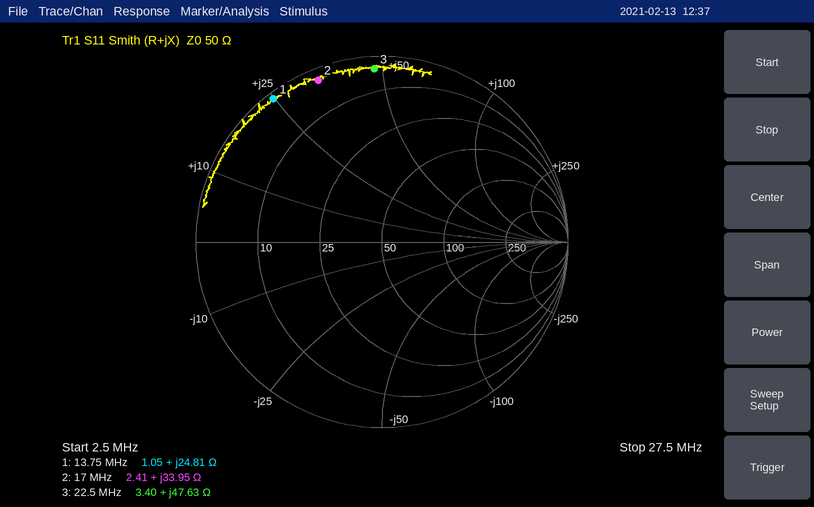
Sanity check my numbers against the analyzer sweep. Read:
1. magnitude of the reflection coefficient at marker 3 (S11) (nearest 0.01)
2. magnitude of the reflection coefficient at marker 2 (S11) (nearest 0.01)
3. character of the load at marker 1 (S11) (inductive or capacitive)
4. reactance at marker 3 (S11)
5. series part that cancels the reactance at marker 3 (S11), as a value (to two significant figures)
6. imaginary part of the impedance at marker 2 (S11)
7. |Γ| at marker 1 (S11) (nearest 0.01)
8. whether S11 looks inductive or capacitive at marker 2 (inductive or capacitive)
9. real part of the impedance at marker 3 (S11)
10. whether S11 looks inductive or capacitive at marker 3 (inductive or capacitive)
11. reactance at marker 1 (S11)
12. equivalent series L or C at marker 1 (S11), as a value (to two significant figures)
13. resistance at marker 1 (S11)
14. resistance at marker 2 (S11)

0.93
0.94
inductive
+47.63 Ω
150 pF
+33.95 Ω
0.97
inductive
3.40 Ω
inductive
+24.81 Ω
290 nH
1.05 Ω
2.41 Ω
